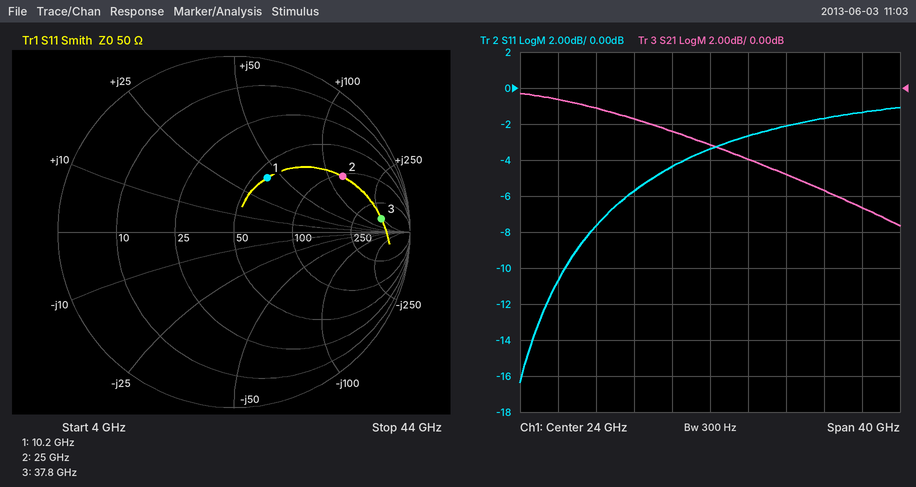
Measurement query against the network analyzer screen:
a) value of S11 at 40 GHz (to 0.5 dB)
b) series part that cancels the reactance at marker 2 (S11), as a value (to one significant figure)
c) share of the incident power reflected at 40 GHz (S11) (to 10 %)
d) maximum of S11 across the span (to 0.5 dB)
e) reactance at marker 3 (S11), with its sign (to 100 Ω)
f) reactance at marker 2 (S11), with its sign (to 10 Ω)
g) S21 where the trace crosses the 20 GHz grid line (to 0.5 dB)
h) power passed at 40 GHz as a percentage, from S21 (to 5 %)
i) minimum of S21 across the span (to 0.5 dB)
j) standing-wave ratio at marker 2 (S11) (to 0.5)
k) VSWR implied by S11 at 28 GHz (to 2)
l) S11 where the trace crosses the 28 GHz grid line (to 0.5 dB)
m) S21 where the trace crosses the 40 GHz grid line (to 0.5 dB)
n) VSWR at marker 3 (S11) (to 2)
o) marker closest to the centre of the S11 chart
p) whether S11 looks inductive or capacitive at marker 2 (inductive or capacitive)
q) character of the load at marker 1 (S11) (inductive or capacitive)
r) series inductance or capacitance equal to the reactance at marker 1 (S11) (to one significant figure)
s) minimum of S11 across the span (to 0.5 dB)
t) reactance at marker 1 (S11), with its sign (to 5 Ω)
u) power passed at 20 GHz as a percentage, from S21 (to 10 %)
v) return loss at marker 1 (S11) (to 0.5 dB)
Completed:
-1.5 dB
50 fF
70 %
-1.0 dB
+200 Ω
+130 Ω
-2.5 dB
20 %
-7.5 dB
5.5
6
-2.5 dB
-6.5 dB
12
marker 1
inductive
inductive
600 pH
-16.5 dB
+40 Ω
60 %
9.0 dB
